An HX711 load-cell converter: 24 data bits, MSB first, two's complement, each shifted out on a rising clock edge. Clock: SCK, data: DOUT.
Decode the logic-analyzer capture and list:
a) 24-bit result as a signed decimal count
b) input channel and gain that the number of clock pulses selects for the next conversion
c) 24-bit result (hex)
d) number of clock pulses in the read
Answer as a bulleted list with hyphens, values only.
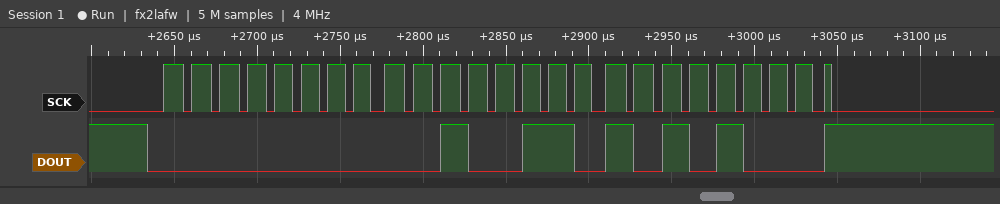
- 9896
- channel A, gain 128
- 0x0026A8
- 25
